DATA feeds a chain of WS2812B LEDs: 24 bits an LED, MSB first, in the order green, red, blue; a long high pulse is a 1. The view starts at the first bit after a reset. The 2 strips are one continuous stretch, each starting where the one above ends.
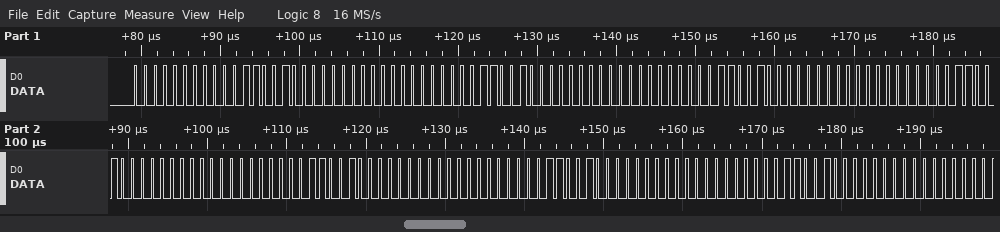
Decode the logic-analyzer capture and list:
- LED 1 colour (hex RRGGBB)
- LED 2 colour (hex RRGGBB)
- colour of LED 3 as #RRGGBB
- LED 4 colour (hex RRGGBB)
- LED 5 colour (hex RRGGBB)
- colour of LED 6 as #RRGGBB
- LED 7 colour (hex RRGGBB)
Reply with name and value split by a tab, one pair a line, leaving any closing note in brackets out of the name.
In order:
LED 1 colour	#190000
LED 2 colour	#190000
colour of LED 3 as #RRGGBB	#190000
LED 4 colour	#190000
LED 5 colour	#190000
colour of LED 6 as #RRGGBB	#190000
LED 7 colour	#190000
